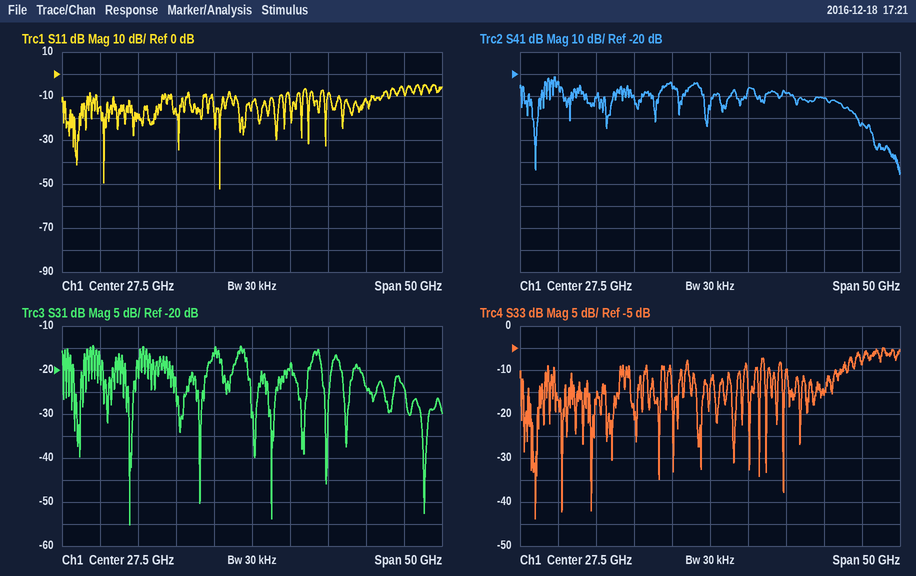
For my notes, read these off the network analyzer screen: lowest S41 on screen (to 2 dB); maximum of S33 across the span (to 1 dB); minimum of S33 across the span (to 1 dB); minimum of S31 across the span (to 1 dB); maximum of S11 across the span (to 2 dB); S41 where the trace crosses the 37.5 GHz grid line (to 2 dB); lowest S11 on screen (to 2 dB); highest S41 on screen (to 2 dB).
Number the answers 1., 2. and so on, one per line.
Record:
1. -66 dB
2. -5 dB
3. -44 dB
4. -55 dB
5. -4 dB
6. -28 dB
7. -52 dB
8. -22 dB
